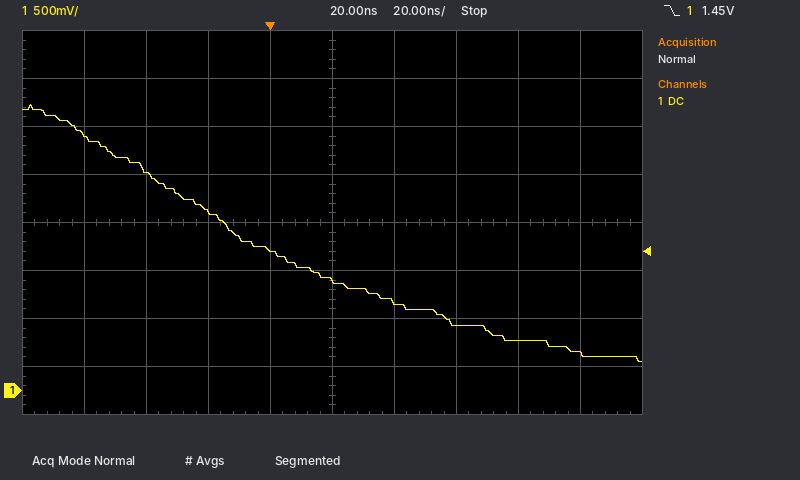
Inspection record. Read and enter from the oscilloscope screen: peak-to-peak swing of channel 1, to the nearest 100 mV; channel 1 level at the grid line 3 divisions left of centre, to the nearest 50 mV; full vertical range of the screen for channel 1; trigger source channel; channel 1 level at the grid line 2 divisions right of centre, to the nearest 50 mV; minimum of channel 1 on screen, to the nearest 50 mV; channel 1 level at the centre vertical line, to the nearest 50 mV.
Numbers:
2.70 V
2.30 V
4 V
channel 1
700 mV
300 mV
1.15 V
